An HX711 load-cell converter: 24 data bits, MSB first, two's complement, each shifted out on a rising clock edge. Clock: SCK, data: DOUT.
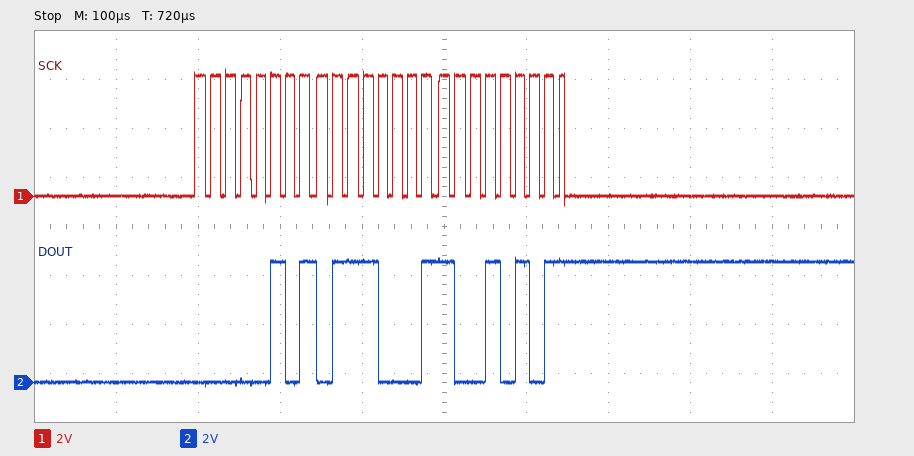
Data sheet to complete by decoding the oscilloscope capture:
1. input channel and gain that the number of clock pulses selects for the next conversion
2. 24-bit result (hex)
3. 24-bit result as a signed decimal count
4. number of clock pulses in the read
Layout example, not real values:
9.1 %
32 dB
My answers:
channel A, gain 128
0x057195
356757
25
